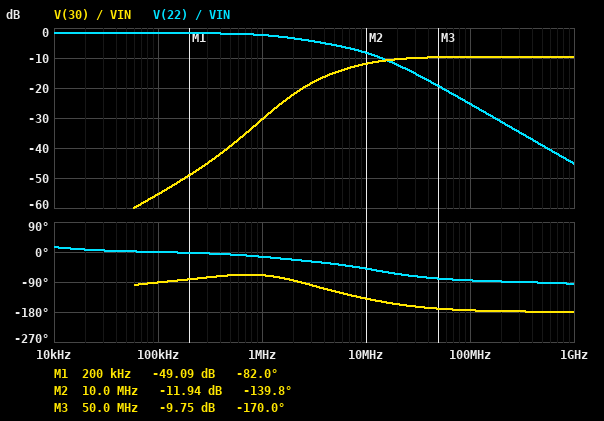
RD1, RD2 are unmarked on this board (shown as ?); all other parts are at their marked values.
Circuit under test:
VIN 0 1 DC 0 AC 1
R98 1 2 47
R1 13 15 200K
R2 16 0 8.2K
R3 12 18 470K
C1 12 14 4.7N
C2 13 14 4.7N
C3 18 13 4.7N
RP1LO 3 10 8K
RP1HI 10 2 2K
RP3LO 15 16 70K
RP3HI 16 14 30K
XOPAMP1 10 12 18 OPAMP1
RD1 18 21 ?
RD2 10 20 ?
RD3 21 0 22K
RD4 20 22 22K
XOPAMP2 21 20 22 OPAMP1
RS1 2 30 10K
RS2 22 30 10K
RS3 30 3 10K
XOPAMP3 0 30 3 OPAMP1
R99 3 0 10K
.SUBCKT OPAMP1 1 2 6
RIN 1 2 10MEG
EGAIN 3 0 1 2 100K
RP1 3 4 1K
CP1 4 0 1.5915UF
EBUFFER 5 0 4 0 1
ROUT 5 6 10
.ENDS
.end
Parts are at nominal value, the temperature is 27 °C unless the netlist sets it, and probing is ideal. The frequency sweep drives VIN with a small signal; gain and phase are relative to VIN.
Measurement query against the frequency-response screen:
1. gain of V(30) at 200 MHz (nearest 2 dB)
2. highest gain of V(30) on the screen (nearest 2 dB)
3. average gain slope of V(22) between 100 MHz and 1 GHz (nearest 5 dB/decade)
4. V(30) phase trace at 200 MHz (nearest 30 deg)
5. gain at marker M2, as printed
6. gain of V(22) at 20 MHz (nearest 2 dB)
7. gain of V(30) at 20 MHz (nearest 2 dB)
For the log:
-10 dB
-10 dB
-20 dB/decade
-180 deg
-11.94 dB
-12 dB
-10 dB
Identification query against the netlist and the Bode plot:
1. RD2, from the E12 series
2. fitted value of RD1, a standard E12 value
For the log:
8.2 kΩ
33 kΩ
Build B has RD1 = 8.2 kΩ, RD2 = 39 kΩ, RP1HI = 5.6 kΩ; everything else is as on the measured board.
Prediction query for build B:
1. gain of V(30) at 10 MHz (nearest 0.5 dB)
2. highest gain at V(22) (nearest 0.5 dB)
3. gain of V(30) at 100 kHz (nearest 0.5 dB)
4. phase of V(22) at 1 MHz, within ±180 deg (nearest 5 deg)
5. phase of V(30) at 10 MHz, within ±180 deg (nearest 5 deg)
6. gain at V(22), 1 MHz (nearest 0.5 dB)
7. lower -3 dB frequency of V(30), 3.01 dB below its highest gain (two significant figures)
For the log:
-11.0 dB
-8.0 dB
-39.5 dB
-165 deg
-170 deg
-19.0 dB
2.5 MHz
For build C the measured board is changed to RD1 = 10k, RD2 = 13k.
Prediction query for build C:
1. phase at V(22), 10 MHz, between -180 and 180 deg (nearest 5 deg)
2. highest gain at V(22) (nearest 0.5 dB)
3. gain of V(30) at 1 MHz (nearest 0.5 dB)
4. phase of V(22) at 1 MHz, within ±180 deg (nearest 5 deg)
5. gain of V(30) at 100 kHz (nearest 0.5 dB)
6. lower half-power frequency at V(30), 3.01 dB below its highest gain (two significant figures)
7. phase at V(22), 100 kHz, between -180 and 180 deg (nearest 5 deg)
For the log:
-15 deg
9.0 dB
-20.0 dB
120 deg
-39.5 dB
11 MHz
160 deg
